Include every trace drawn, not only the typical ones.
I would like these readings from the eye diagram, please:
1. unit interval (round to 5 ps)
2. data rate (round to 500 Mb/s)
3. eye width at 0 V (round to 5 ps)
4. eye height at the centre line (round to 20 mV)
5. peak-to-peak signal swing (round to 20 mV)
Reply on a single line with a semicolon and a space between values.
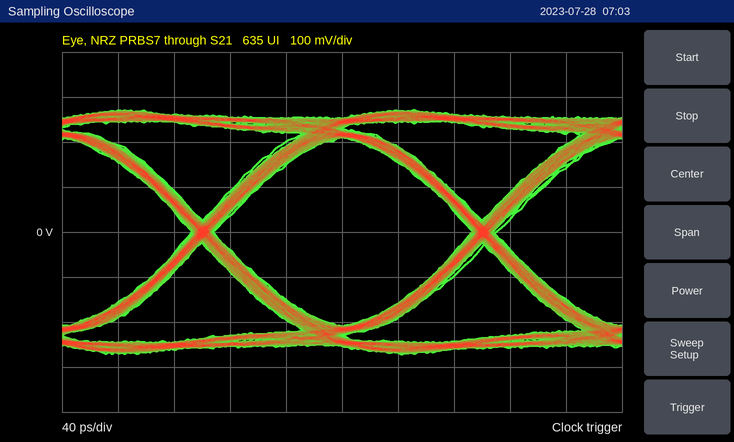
200 ps; 5.0 Gb/s; 185 ps; 420 mV; 540 mV
